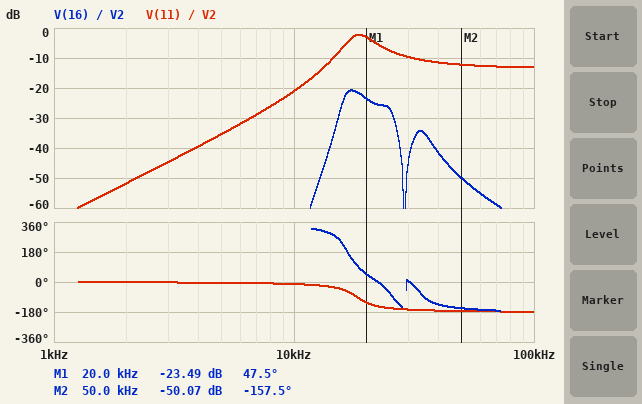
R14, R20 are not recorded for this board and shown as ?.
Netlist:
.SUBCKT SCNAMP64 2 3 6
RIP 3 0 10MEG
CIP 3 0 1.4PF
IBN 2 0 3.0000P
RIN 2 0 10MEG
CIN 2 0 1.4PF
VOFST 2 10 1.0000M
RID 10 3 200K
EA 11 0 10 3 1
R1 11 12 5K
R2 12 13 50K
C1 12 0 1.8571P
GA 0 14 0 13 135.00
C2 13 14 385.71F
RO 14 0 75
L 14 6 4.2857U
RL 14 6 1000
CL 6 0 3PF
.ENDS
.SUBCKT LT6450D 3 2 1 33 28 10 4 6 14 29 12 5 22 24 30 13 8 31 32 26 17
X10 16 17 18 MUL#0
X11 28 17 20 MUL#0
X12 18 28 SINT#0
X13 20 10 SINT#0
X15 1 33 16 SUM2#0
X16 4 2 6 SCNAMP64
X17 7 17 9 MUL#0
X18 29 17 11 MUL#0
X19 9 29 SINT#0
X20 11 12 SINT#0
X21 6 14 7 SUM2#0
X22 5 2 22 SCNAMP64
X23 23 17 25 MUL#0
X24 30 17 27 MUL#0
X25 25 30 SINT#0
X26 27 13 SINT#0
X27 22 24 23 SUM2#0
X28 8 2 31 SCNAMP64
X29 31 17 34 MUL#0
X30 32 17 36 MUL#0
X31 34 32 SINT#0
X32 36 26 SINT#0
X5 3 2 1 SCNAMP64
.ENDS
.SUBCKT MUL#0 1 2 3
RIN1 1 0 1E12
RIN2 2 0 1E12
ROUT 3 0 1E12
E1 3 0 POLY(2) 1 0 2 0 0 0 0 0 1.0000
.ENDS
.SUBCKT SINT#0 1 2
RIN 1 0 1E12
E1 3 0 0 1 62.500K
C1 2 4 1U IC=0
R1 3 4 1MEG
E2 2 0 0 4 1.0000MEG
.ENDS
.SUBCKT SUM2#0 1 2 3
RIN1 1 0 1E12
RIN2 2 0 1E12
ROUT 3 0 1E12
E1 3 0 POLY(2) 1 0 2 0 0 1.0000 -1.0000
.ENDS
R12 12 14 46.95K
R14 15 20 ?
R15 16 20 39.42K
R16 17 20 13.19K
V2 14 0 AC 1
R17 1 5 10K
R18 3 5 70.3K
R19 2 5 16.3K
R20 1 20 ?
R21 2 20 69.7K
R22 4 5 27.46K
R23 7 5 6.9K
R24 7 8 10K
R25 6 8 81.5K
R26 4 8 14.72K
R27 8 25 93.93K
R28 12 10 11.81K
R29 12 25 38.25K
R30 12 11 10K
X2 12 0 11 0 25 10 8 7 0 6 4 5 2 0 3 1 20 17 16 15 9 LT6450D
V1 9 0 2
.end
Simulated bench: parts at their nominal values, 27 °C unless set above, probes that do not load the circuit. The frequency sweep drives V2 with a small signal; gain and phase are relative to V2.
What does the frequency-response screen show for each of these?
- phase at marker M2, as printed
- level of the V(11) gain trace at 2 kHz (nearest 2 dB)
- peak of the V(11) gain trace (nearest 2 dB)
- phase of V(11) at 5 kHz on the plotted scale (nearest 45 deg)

-157.5 deg
-52 dB
-2 dB
0 deg
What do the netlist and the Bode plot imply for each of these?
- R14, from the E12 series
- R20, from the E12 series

4.7 kΩ
33 kΩ
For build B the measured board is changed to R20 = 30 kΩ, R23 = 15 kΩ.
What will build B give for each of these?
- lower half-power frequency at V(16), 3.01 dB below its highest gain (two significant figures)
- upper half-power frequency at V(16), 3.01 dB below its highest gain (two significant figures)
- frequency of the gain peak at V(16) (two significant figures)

17 kHz
26 kHz
19 kHz
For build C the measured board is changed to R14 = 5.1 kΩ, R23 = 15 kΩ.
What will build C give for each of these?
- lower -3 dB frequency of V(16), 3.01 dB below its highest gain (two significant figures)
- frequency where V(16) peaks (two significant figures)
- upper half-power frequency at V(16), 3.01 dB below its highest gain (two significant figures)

17 kHz
19 kHz
26 kHz
